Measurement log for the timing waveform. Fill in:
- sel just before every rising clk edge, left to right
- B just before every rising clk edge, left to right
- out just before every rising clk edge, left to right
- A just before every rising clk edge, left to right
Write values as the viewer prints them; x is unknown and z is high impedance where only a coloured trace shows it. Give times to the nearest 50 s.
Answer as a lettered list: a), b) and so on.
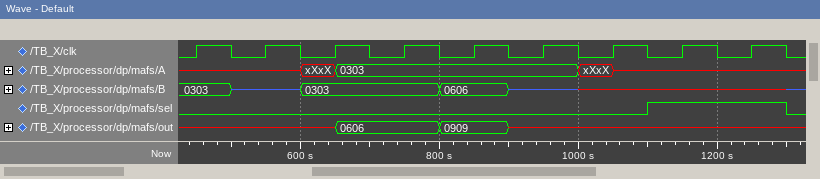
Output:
a) 0 0 0 0 0 0 0 1 1
b) 0303, z, 0303, 0303, 0606, z, x, x, x
c) x, x, x, 0606, 0909, x, x, x, x
d) x, x, xXxX, 0303, 0303, 0303, xXxX, x, x
